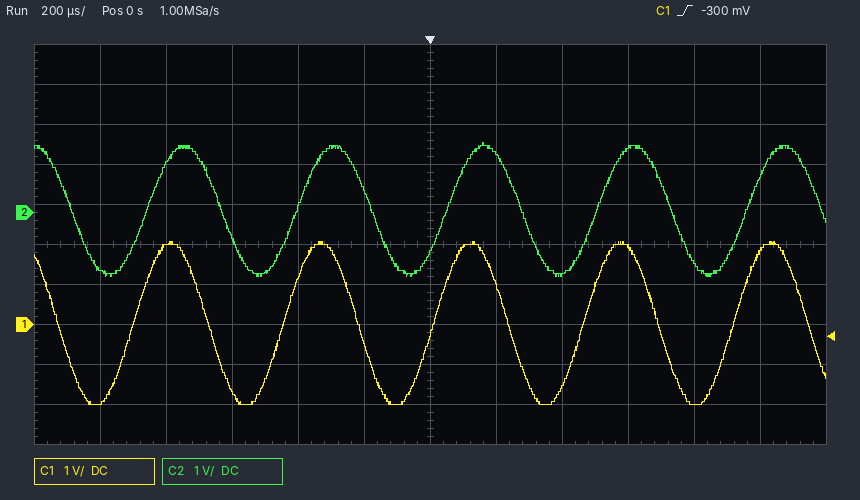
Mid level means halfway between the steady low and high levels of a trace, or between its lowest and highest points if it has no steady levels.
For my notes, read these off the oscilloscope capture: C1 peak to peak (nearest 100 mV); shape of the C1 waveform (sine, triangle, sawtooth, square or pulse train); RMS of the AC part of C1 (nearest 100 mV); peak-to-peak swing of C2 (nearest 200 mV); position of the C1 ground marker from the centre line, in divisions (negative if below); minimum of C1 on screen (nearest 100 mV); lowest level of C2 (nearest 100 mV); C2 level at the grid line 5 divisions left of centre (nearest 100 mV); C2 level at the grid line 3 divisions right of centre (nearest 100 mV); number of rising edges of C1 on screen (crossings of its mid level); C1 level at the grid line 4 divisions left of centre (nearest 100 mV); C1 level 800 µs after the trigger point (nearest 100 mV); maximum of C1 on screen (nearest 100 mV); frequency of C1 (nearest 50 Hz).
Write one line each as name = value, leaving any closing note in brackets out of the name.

C1 peak to peak = 4.1 V
shape of the C1 waveform = sine
RMS of the AC part of C1 = 1.4 V
peak-to-peak swing of C2 = 3.4 V
position of the C1 ground marker from the centre line, in divisions = -2.0 div
minimum of C1 on screen = -2.0 V
lowest level of C2 = -1.6 V
C2 level at the grid line 5 divisions left of centre = -1.4 V
C2 level at the grid line 3 divisions right of centre = 1.6 V
number of rising edges of C1 on screen = 5
C1 level at the grid line 4 divisions left of centre = 2.0 V
C1 level 800 µs after the trigger point = -2.0 V
maximum of C1 on screen = 2.1 V
frequency of C1 = 2.20 kHz
